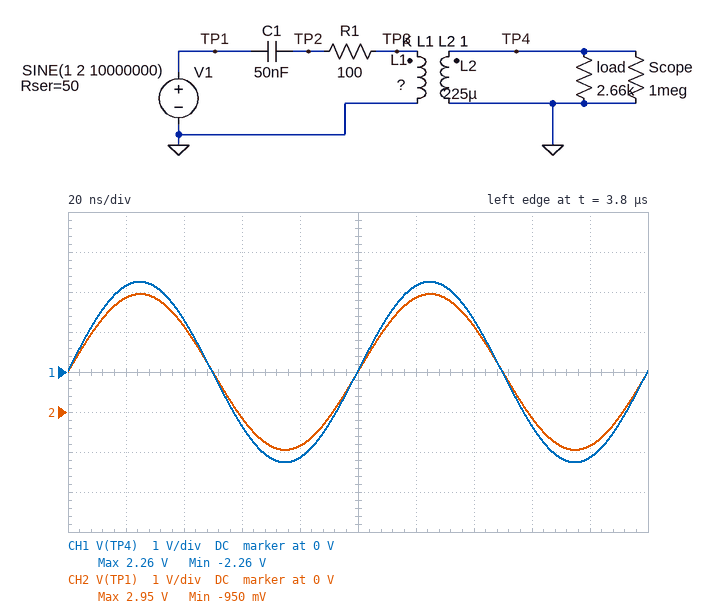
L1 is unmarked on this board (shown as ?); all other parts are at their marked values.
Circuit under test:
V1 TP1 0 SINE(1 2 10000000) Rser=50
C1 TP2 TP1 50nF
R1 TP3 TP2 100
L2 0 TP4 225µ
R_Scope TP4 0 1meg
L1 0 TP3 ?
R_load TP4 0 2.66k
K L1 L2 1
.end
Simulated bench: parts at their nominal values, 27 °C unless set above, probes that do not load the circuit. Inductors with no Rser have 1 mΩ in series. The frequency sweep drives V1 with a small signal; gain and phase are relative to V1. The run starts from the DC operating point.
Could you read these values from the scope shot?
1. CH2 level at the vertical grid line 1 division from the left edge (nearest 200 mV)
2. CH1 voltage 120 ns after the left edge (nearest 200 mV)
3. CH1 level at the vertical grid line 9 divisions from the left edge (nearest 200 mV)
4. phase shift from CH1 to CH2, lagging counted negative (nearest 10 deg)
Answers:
2.8 V
2.2 V
-2.2 V
0 deg
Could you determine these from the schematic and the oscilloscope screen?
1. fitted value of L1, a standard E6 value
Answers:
150 µH
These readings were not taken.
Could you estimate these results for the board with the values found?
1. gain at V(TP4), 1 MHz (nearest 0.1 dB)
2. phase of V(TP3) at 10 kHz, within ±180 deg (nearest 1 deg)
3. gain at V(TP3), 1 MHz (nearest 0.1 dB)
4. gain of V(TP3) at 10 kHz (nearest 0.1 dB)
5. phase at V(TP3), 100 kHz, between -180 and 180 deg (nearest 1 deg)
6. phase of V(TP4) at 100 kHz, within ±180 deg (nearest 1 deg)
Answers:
1.0 dB
154 deg
-0.8 dB
-31.2 dB
65 deg
65 deg
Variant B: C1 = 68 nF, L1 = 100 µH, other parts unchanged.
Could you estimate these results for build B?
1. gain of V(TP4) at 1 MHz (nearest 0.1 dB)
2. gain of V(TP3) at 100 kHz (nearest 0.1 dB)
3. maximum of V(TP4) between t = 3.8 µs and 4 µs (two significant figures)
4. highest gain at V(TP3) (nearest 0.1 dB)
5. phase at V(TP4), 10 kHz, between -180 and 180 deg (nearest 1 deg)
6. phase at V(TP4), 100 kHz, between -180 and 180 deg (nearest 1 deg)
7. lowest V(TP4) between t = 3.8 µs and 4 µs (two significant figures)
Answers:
2.3 dB
-8.0 dB
2.7 V
-1.0 dB
146 deg
73 deg
-2.7 V
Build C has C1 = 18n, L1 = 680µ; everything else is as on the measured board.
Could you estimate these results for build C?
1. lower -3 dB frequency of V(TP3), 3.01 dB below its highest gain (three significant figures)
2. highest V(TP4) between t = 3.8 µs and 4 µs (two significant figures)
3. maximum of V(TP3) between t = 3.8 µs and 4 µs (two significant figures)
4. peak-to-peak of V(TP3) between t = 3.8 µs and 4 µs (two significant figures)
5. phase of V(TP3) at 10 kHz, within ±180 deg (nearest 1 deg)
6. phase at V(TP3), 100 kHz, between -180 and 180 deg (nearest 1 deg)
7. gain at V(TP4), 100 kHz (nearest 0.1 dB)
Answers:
37.9 kHz
1.1 V
2.0 V
3.9 V
170 deg
24 deg
-3.8 dB
